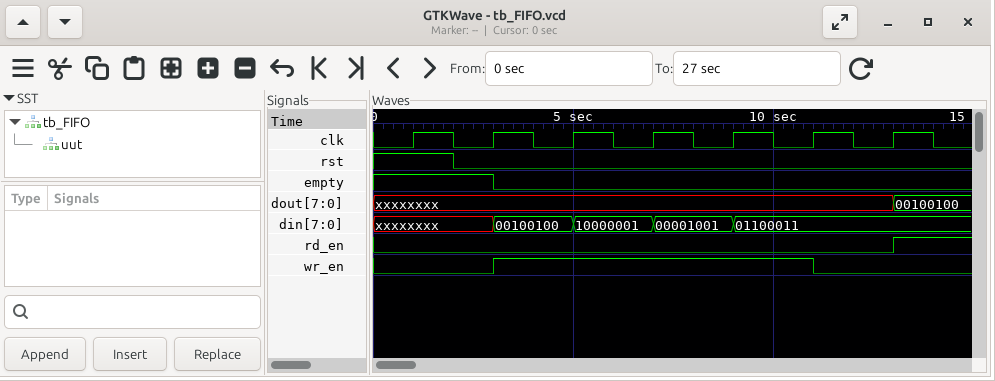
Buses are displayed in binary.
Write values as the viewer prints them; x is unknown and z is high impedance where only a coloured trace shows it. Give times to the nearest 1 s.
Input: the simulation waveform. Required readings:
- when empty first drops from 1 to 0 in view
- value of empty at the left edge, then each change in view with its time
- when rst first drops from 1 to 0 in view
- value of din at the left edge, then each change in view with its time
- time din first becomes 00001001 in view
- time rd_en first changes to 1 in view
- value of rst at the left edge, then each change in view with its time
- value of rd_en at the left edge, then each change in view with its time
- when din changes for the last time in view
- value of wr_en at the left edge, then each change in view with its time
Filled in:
3 s
1, 0 at 3 s
2 s
xxxxxxxx, 00100100 at 3 s, 10000001 at 5 s, 00001001 at 7 s, 01100011 at 9 s
7 s
13 s
1, 0 at 2 s
0, 1 at 13 s
9 s
0, 1 at 3 s, 0 at 11 s
